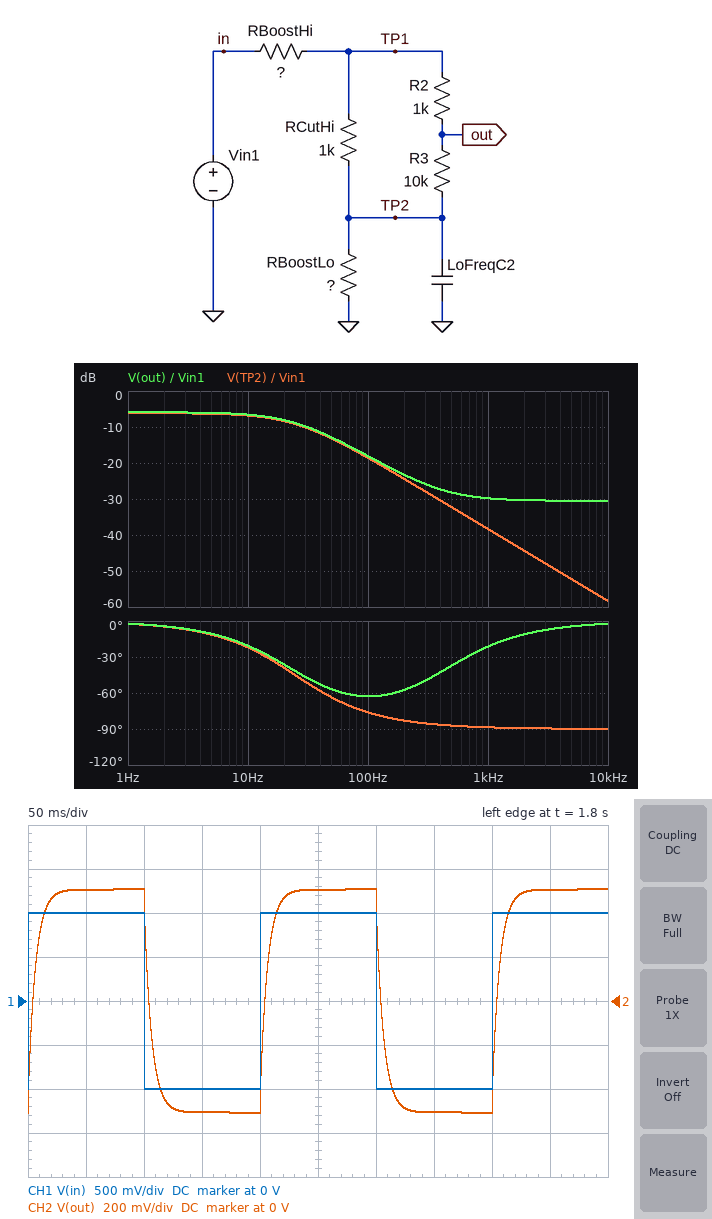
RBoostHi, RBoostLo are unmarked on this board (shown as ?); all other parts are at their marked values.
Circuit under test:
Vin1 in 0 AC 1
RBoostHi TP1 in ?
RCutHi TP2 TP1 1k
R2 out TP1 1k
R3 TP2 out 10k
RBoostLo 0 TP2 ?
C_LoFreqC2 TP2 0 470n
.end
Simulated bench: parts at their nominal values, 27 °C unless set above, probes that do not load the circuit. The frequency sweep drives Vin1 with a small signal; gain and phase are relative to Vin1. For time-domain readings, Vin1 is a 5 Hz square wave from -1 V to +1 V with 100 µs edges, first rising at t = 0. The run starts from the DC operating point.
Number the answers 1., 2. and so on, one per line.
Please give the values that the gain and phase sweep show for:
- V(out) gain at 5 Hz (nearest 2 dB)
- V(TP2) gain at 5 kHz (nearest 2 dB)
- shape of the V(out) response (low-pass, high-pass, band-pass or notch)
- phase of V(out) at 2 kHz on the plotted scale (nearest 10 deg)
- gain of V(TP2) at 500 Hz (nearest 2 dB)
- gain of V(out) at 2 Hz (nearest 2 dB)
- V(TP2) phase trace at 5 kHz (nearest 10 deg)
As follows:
1. -6 dB
2. -52 dB
3. low-pass
4. -10 deg
5. -32 dB
6. -6 dB
7. -90 deg
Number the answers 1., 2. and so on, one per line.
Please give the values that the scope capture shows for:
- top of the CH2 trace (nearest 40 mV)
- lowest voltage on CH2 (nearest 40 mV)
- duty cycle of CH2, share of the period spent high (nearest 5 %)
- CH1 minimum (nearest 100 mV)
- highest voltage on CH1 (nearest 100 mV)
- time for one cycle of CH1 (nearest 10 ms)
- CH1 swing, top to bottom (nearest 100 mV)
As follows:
1. 520 mV
2. -520 mV
3. 50 %
4. -1.0 V
5. 1.0 V
6. 200 ms
7. 2.0 V
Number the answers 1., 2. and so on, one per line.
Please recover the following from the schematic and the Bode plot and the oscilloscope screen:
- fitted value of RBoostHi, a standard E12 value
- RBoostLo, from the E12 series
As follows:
1. 27 kΩ
2. 27 kΩ
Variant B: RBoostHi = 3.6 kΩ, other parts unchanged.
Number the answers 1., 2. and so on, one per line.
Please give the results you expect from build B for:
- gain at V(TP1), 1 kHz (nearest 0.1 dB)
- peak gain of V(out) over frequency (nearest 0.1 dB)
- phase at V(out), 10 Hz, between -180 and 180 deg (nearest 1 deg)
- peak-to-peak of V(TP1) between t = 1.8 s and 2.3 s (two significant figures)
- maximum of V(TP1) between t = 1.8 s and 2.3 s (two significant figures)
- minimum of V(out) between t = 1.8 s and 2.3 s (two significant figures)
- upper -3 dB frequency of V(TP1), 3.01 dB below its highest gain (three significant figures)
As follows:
1. -13.3 dB
2. -1.1 dB
3. -5 deg
4. 1.8 V
5. 890 mV
6. -880 mV
7. 92.5 Hz
